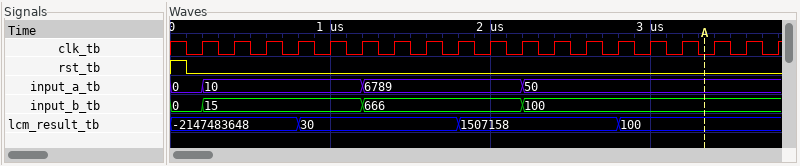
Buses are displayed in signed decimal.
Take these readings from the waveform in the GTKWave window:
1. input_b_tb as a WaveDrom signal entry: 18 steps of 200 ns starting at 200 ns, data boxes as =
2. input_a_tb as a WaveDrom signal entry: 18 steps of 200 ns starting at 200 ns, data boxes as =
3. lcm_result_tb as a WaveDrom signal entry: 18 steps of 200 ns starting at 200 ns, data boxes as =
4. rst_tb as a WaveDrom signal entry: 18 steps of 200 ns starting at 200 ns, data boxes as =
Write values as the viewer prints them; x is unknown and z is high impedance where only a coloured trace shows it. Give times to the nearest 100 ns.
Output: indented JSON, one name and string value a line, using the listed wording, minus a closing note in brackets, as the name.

{
  "input_b_tb as a WaveDrom signal entry: 18 steps of 200 ns starting at 200 ns, data boxes as =": "{name: 'input_b_tb', wave: '=....=....=.......', data: '15 666 100'}",
  "input_a_tb as a WaveDrom signal entry: 18 steps of 200 ns starting at 200 ns, data boxes as =": "{name: 'input_a_tb', wave: '=....=....=.......', data: '10 6789 50'}",
  "lcm_result_tb as a WaveDrom signal entry: 18 steps of 200 ns starting at 200 ns, data boxes as =": "{name: 'lcm_result_tb', wave: '=..=....=....=....', data: '-2147483648 30 1507158 100'}",
  "rst_tb as a WaveDrom signal entry: 18 steps of 200 ns starting at 200 ns, data boxes as =": "{name: 'rst_tb', wave: '0.................'}"
}
